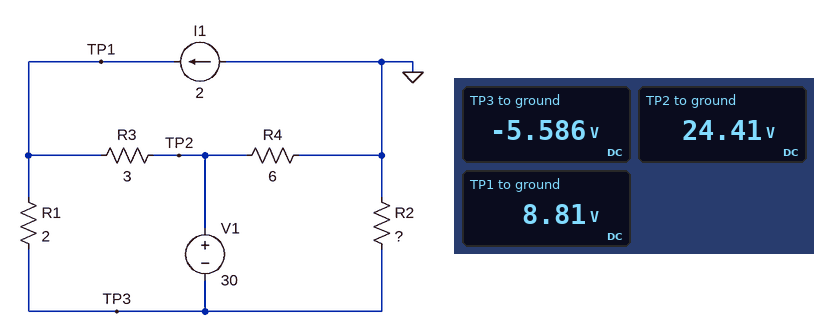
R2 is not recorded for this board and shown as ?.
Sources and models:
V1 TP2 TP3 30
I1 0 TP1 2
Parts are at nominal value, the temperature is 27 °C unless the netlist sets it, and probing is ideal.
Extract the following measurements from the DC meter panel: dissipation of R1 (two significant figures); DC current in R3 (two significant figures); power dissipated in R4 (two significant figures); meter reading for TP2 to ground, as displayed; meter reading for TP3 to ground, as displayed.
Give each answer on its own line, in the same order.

100 W
5.2 A
99 W
24.41 V
-5.586 V
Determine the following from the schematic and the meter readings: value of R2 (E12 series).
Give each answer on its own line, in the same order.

2.7 Ω
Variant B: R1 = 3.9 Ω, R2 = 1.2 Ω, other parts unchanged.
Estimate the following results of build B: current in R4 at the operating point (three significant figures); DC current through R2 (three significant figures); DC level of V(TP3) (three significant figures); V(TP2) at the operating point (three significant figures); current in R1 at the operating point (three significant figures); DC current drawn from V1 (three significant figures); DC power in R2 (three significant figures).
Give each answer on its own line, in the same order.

4.50 A
2.50 A
-3.00 V
27.0 V
5.22 A
7.72 A
7.50 W
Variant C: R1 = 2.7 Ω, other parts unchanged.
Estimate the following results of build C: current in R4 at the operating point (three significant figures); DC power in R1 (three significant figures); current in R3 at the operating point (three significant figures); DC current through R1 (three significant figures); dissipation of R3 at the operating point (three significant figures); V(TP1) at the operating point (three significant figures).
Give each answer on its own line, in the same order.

4.07 A
108 W
4.32 A
6.32 A
55.9 W
11.5 V
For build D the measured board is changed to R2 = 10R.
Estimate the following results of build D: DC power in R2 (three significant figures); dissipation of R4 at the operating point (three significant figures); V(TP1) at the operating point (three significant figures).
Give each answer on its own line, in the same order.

12.7 W
58.6 W
3.15 V
